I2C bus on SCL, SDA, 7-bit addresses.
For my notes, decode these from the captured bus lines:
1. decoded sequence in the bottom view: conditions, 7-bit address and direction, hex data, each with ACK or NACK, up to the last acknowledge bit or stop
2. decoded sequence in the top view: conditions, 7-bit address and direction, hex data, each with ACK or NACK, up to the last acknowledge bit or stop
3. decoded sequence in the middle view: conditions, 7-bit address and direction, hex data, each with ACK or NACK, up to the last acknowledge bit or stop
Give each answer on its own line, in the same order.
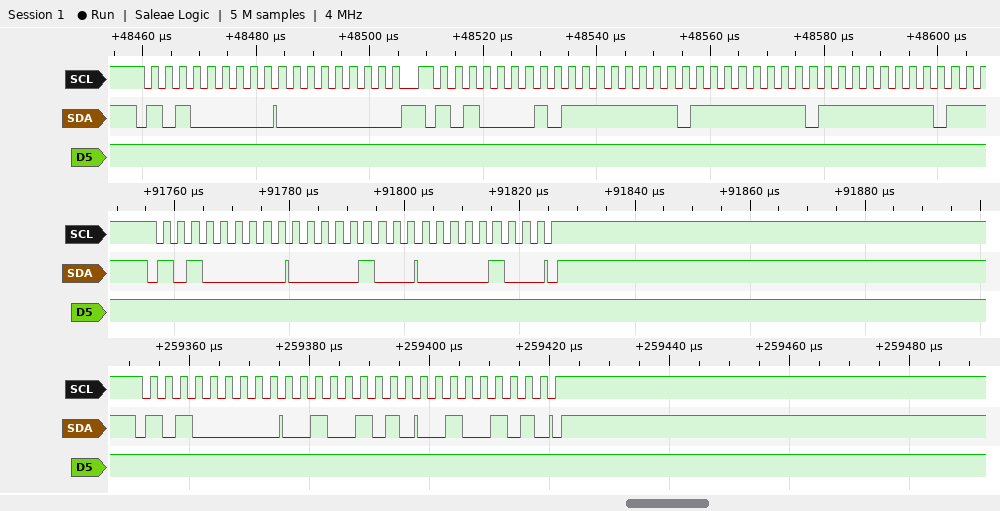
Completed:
start, address 50 write ACK, 25 ACK, 25 ACK, stop
start, address 50 write ACK, 00 ACK, repeated start, address 50 read ACK, FF ACK, FF ACK, FF ACK
start, address 50 write ACK, 04 ACK, 04 ACK, stop
